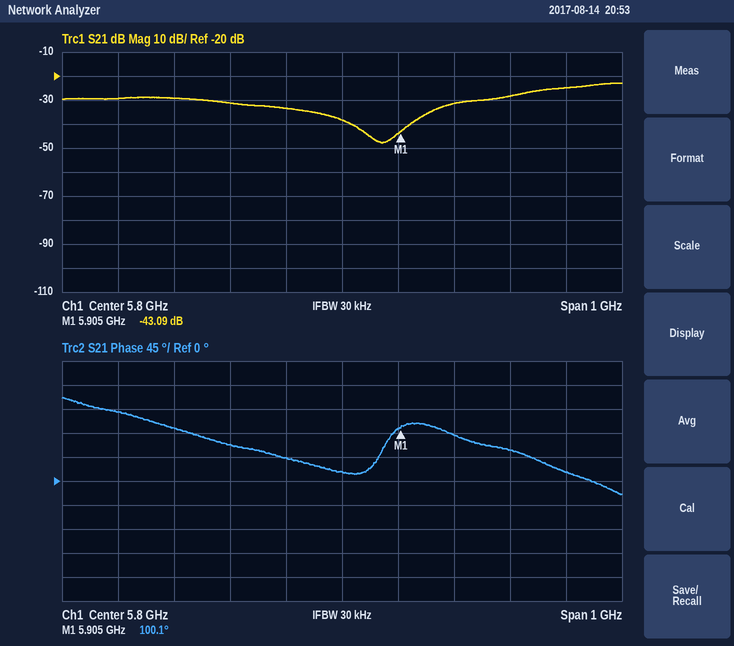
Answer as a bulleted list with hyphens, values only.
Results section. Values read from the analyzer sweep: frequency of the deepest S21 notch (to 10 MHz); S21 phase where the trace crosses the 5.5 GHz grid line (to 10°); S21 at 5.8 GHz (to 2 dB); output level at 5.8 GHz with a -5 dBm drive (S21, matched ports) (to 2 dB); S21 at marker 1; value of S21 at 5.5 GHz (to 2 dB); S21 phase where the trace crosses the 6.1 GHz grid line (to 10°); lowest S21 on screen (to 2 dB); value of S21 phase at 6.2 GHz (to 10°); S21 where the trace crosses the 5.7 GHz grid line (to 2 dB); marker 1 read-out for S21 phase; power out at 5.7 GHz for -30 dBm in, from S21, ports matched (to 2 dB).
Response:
- 5.87 GHz
- 100°
- -38 dB
- -44 dBm
- -43.09 dB
- -30 dB
- 60°
- -48 dB
- 20°
- -34 dB
- 100.1°
- -64 dBm
